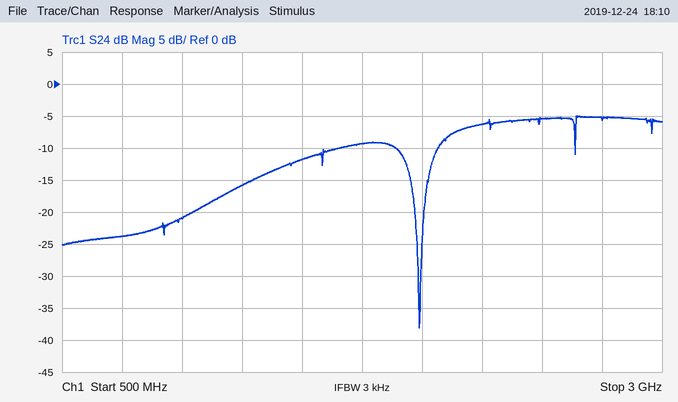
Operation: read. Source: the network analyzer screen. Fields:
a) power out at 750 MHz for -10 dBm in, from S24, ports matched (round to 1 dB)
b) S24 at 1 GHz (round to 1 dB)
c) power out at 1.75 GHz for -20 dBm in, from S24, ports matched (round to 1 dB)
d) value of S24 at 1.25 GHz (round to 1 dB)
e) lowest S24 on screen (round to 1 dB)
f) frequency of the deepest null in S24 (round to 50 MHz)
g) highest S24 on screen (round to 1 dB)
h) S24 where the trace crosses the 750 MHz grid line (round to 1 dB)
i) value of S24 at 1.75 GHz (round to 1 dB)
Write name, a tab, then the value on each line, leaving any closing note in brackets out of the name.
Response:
power out at 750 MHz for -10 dBm in, from S24, ports matched	-34 dBm
S24 at 1 GHz	-21 dB
power out at 1.75 GHz for -20 dBm in, from S24, ports matched	-29 dBm
value of S24 at 1.25 GHz	-16 dB
lowest S24 on screen	-38 dB
frequency of the deepest null in S24	2.00 GHz
highest S24 on screen	-5 dB
S24 where the trace crosses the 750 MHz grid line	-24 dB
value of S24 at 1.75 GHz	-9 dB
